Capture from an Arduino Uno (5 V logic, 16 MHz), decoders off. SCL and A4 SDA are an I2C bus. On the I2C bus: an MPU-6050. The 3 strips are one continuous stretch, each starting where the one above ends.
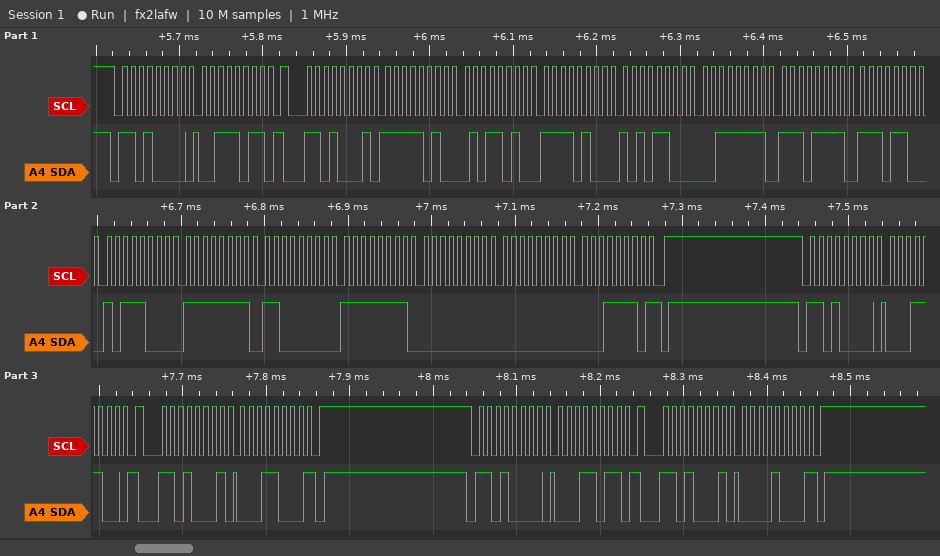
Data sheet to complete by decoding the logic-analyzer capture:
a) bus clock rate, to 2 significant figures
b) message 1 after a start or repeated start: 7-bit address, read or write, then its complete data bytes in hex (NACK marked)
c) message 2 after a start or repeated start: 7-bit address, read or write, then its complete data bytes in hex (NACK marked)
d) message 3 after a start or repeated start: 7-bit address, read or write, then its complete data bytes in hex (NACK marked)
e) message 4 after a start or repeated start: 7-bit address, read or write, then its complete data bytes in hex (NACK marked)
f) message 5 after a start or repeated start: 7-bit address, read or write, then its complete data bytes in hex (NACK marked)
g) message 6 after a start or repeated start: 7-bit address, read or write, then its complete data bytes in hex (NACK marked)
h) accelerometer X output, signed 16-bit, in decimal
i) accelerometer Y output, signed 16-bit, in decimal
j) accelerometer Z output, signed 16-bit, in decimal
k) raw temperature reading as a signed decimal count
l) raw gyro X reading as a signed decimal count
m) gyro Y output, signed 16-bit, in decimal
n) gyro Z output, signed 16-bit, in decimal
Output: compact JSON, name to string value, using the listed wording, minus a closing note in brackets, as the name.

{"bus clock rate, to 2 significant figures": "100 kHz", "message 1 after a start or repeated start: 7-bit address, read or write, then its complete data bytes in hex": "0x68 write: 3B", "message 2 after a start or repeated start: 7-bit address, read or write, then its complete data bytes in hex": "0x68 read: FA 5A F4 AC 3F EF EC B8 FF C0 FF 00 00 1E NACK", "message 3 after a start or repeated start: 7-bit address, read or write, then its complete data bytes in hex": "0x68 write: 1C", "message 4 after a start or repeated start: 7-bit address, read or write, then its complete data bytes in hex": "0x68 read: 18 NACK", "message 5 after a start or repeated start: 7-bit address, read or write, then its complete data bytes in hex": "0x68 write: 1B", "message 6 after a start or repeated start: 7-bit address, read or write, then its complete data bytes in hex": "0x68 read: 08 NACK", "accelerometer X output, signed 16-bit, in decimal": "-1446", "accelerometer Y output, signed 16-bit, in decimal": "-2900", "accelerometer Z output, signed 16-bit, in decimal": "16367", "raw temperature reading as a signed decimal count": "-4936", "raw gyro X reading as a signed decimal count": "-64", "gyro Y output, signed 16-bit, in decimal": "-256", "gyro Z output, signed 16-bit, in decimal": "30"}
